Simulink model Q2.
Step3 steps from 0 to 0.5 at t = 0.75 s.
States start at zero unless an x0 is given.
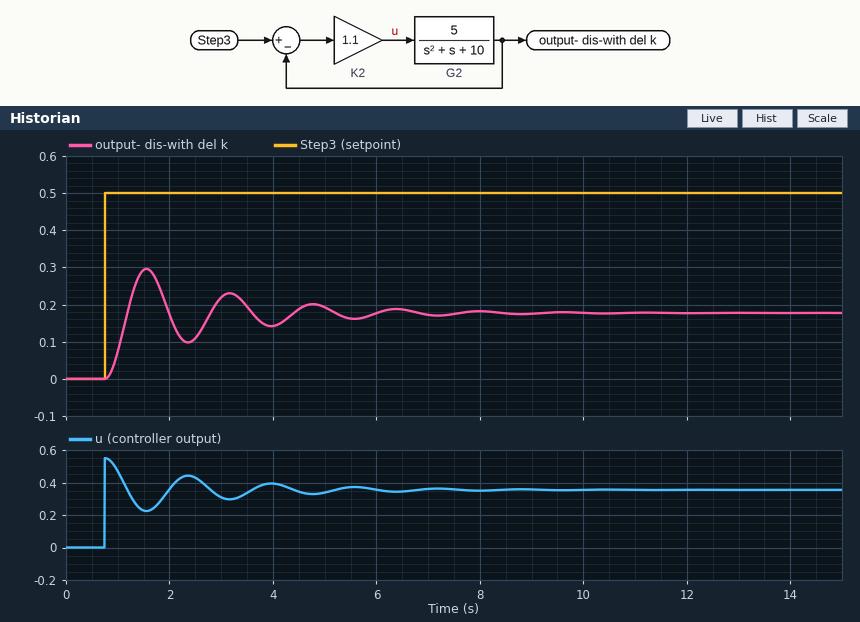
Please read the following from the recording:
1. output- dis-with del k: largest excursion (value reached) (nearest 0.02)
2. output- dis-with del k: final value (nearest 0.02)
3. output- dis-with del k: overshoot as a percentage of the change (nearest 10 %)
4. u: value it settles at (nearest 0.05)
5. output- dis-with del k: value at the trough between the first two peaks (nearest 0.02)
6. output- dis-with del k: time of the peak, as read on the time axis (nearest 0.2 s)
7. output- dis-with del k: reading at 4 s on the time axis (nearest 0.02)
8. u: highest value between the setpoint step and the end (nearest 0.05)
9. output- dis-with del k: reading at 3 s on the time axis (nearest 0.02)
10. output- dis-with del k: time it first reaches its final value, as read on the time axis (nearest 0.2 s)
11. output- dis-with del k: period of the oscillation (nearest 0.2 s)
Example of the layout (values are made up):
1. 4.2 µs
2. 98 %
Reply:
1. 0.30
2. 0.18
3. 70 %
4. 0.35
5. 0.10
6. 1.6 s
7. 0.14
8. 0.55
9. 0.22
10. 1.2 s
11. 1.6 s
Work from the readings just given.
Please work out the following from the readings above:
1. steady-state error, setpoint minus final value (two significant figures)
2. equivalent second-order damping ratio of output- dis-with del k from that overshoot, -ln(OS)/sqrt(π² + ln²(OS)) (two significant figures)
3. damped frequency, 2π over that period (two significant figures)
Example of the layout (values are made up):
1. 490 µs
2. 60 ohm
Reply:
1. 0.32
2. 0.11
3. 3.9 rad/s
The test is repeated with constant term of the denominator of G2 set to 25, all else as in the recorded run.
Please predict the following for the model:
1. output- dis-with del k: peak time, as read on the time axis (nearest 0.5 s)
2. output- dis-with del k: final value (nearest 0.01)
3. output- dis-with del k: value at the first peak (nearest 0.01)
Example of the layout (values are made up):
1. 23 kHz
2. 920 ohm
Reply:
1. 1.5 s
2. 0.09
3. 0.16
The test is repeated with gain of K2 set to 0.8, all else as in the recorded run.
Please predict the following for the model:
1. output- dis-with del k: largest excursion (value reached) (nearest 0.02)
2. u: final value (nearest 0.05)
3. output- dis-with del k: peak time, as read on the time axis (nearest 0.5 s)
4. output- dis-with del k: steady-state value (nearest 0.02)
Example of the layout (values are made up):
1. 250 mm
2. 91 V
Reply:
1. 0.24
2. 0.30
3. 1.5 s
4. 0.14
